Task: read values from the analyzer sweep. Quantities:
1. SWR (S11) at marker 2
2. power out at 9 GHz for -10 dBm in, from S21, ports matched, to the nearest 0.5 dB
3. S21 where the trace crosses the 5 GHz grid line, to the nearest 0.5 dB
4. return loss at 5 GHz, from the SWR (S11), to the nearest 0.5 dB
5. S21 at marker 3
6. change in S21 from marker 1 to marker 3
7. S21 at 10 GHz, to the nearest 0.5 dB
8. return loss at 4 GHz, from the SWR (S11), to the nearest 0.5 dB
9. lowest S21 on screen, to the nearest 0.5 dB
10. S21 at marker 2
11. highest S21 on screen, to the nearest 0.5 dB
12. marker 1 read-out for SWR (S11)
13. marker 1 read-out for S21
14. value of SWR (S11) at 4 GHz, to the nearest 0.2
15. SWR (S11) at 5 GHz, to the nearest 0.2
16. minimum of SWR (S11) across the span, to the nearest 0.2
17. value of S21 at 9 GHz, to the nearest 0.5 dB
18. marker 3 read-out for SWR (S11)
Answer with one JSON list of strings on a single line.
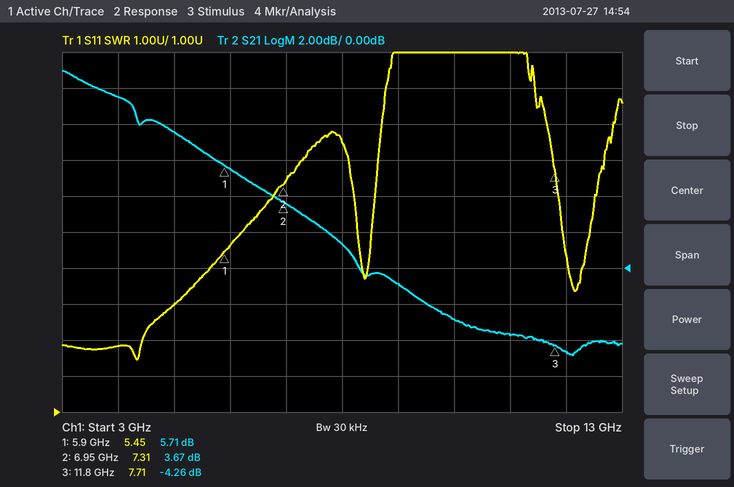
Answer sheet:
["7.31", "-11.0 dBm", "7.5 dB", "4.5 dB", "-4.26 dB", "-9.97 dB", "-3.0 dB", "6.5 dB", "-5.0 dB", "3.67 dB", "11.0 dB", "5.45", "5.71 dB", "2.8", "4.0", "2.4", "-1.0 dB", "7.71"]
